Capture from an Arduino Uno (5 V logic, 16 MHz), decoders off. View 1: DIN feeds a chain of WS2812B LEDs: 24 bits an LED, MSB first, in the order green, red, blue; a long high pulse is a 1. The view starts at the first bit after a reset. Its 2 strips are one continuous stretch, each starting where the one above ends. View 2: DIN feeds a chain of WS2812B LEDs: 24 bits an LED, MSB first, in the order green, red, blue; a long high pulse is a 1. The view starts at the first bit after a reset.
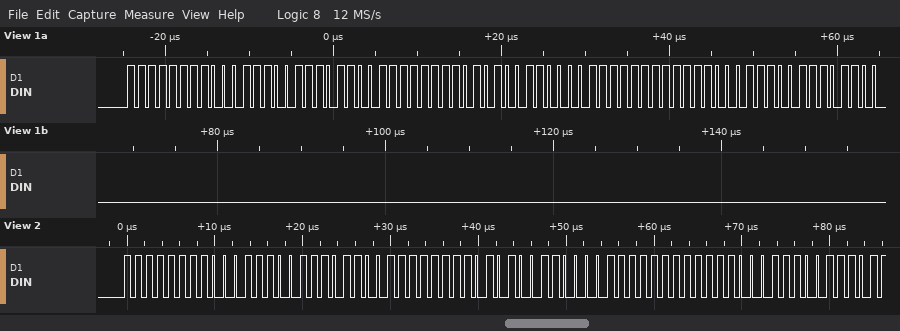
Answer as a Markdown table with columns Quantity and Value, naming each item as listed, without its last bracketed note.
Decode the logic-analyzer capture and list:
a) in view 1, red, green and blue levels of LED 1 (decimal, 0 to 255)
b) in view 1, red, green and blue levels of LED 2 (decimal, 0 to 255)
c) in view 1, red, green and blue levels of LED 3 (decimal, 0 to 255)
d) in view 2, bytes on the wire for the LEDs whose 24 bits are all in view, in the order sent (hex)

| Quantity | Value |
|---|---|
| in view 1, red, green and blue levels of LED 1 | 28, 255, 236 |
| in view 1, red, green and blue levels of LED 2 | 83, 255, 15 |
| in view 1, red, green and blue levels of LED 3 | 28, 255, 236 |
| in view 2, bytes on the wire for the LEDs whose 24 bits are all in view, in the order sent | FF 1C EC FF 53 0F |
